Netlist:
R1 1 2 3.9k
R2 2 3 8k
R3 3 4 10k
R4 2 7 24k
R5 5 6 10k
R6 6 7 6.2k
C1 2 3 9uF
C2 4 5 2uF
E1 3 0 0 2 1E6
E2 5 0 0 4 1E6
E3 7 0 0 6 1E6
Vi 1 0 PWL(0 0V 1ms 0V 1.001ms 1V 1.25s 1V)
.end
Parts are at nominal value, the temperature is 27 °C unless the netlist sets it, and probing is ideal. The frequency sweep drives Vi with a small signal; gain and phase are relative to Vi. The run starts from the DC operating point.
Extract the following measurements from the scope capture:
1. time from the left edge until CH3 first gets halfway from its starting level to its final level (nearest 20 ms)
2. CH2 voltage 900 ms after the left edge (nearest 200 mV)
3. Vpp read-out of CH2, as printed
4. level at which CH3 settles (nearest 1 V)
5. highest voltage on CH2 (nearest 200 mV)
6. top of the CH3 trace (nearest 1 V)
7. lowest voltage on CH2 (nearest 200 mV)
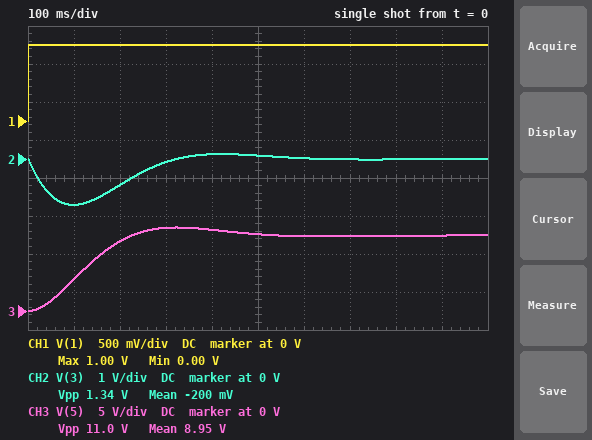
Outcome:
120 ms
0 V
1.34 V
10 V
200 mV
11 V
-1.2 V
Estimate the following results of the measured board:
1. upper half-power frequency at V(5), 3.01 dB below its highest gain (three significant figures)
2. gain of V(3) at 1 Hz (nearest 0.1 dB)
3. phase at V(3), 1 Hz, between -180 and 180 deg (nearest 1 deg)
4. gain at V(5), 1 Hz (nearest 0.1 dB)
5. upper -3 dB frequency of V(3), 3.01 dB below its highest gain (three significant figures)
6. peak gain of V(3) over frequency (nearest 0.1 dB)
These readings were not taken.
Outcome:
2.15 Hz
2.4 dB
-130 deg
20.4 dB
3.31 Hz
6.2 dB
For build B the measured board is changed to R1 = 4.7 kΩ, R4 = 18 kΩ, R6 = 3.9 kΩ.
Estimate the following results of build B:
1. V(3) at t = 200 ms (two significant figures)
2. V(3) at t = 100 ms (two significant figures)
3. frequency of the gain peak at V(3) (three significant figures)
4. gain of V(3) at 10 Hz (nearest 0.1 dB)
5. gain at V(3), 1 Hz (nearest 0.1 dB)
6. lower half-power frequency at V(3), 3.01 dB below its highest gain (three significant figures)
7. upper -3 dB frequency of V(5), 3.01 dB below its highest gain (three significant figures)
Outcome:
-690 mV
-1.0 V
1.75 Hz
-8.4 dB
1.9 dB
961 mHz
1.90 Hz
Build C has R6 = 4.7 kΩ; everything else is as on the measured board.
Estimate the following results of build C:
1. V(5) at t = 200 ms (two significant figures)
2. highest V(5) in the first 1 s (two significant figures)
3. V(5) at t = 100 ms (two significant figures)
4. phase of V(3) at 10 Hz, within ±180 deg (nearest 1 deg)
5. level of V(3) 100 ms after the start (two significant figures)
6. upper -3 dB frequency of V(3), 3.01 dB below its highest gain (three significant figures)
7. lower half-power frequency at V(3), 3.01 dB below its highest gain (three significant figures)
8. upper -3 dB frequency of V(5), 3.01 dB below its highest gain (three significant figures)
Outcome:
10 V
14 V
4.3 V
103 deg
-1.3 V
3.10 Hz
889 mHz
1.75 Hz
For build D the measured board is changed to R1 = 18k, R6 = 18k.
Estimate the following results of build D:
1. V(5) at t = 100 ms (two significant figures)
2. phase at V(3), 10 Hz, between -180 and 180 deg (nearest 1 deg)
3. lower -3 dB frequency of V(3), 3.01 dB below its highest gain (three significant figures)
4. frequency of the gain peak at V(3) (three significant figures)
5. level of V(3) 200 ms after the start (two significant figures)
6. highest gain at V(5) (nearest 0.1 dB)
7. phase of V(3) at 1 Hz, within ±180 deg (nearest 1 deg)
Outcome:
730 mV
104 deg
2.33 Hz
3.25 Hz
51 mV
1.3 dB
-103 deg
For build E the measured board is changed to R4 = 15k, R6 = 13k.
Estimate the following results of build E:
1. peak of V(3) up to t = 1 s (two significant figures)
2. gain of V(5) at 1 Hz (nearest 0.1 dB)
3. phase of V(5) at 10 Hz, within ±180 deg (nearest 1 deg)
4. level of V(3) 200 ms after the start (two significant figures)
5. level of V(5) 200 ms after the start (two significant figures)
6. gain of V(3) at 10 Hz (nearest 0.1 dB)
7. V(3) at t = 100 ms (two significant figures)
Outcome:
300 mV
10.0 dB
-166 deg
290 mV
3.6 V
-6.0 dB
-610 mV
